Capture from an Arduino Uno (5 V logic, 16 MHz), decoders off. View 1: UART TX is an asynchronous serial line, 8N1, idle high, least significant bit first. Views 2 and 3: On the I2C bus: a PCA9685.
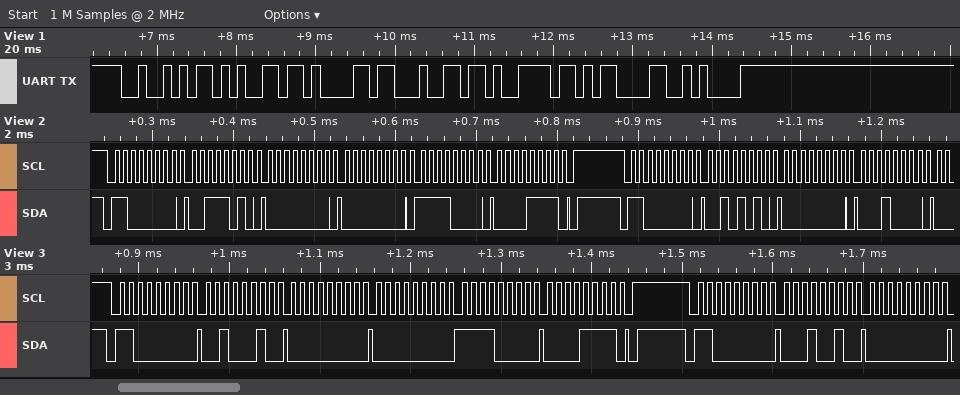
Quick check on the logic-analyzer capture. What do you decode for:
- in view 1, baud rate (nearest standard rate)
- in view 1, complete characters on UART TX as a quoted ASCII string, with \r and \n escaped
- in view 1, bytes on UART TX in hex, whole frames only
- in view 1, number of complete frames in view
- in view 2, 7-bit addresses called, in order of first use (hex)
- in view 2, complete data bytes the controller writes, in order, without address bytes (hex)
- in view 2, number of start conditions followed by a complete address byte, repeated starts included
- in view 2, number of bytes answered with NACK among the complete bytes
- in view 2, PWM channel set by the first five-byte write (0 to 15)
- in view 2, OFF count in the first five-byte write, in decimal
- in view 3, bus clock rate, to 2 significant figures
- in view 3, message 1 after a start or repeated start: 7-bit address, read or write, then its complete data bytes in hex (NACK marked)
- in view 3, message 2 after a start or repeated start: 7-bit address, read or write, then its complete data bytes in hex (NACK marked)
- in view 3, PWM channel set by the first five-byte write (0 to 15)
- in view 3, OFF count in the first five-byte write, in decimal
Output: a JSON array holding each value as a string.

["9600 baud", "\"Ready\\r\\n\"", "0x52 0x65 0x61 0x64 0x79 0x0D 0x0A", "7", "0x60", "3A 00 00 F0 0F 2A 00 10", "2", "0", "13", "4080", "100 kHz", "0x60 write: 22 00 00 F0 0F", "0x60 write: 12 00", "7", "4080"]
